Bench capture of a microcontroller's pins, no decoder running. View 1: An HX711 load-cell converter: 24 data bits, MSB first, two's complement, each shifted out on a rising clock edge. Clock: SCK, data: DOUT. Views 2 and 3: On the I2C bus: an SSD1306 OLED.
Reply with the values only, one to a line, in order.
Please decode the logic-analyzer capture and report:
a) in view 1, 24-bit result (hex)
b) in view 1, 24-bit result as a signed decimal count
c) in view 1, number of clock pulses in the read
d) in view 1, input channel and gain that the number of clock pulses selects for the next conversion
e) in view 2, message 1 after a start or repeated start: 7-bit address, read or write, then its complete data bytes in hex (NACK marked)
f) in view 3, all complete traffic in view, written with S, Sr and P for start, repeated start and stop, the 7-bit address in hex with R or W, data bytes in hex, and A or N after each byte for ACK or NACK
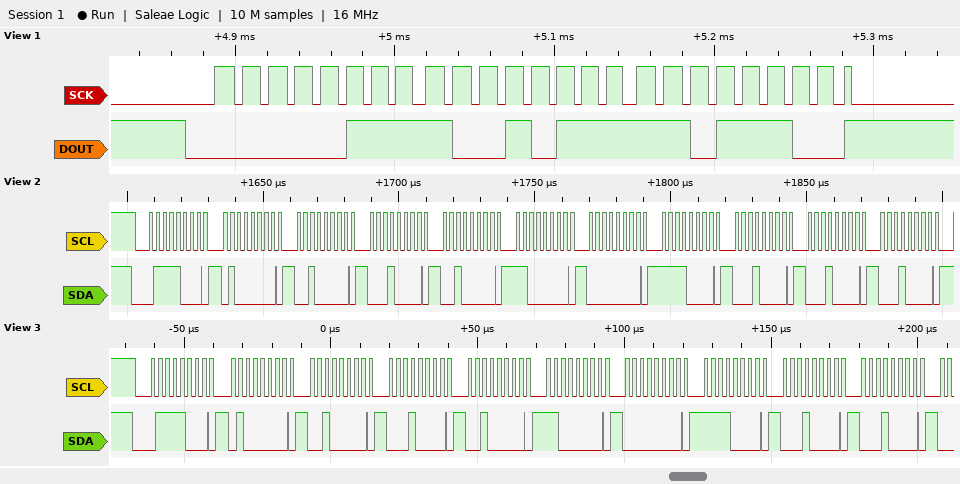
0x0797DC
497628
25
channel A, gain 128
0x3C write: 40 20 10 20 C0 00 F0 10 10 10
S 3CW A 40 A 20 A 10 A 20 A C0 A 00 A F0 A 10 A 10 A
